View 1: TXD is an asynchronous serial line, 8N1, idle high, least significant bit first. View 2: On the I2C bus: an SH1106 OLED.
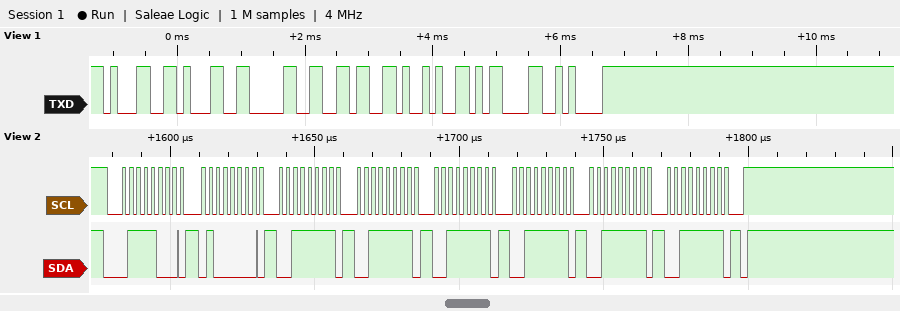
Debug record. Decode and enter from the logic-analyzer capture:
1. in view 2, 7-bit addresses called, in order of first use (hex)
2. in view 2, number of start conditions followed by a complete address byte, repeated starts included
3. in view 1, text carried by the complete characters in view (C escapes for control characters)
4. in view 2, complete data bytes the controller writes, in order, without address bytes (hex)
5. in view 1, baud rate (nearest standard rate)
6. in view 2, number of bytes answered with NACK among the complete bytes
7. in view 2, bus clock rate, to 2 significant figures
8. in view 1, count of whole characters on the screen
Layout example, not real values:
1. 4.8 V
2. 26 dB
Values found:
1. 0x3C
2. 1
3. "1106)\r\n"
4. 40 3F 3F 3F 3F 3F 3F
5. 9600 baud
6. 0
7. 400 kHz
8. 7
